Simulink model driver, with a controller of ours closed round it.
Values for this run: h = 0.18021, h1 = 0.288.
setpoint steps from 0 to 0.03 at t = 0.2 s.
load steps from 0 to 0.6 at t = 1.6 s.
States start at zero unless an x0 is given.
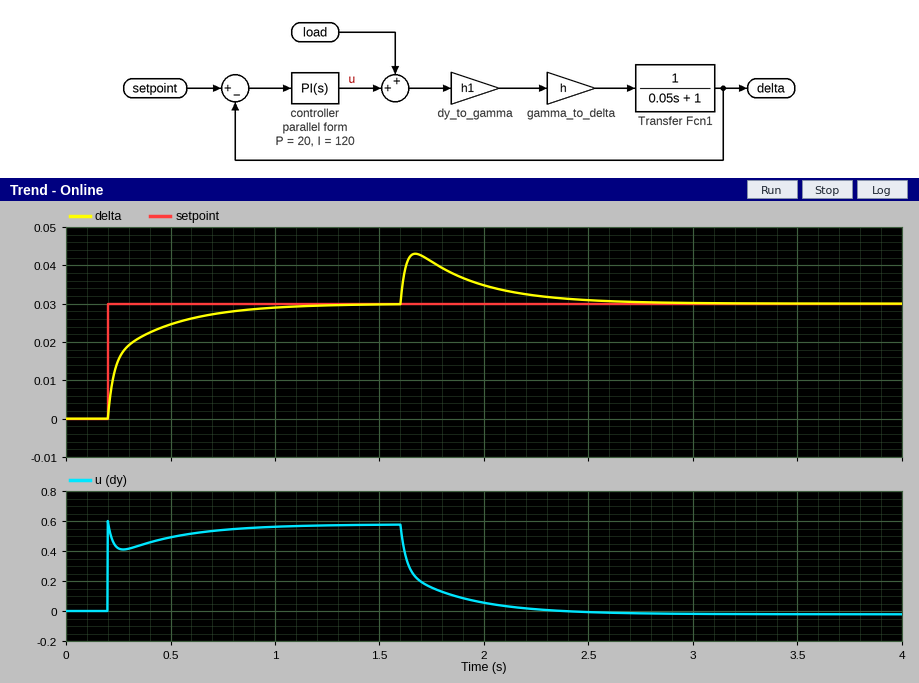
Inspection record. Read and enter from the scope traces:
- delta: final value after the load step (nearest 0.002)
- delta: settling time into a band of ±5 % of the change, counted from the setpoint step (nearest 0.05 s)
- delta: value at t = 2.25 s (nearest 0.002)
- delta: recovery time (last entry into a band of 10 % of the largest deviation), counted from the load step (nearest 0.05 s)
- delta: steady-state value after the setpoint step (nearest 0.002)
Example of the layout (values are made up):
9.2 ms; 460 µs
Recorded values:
0.030; 0.70 s; 0.032; 0.80 s; 0.030
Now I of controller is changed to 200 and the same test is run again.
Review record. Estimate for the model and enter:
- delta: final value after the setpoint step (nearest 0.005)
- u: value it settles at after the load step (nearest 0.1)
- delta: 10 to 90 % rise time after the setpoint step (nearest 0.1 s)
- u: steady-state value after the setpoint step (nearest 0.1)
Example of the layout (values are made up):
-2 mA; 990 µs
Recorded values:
0.030; 0.0; 0.3 s; 0.6
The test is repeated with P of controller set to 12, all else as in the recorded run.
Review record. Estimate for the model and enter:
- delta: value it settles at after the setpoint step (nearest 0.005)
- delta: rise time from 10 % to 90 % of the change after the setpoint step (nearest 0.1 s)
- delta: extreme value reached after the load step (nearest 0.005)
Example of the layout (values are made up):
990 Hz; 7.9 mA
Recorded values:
0.030; 0.4 s; 0.045
